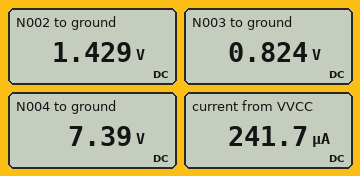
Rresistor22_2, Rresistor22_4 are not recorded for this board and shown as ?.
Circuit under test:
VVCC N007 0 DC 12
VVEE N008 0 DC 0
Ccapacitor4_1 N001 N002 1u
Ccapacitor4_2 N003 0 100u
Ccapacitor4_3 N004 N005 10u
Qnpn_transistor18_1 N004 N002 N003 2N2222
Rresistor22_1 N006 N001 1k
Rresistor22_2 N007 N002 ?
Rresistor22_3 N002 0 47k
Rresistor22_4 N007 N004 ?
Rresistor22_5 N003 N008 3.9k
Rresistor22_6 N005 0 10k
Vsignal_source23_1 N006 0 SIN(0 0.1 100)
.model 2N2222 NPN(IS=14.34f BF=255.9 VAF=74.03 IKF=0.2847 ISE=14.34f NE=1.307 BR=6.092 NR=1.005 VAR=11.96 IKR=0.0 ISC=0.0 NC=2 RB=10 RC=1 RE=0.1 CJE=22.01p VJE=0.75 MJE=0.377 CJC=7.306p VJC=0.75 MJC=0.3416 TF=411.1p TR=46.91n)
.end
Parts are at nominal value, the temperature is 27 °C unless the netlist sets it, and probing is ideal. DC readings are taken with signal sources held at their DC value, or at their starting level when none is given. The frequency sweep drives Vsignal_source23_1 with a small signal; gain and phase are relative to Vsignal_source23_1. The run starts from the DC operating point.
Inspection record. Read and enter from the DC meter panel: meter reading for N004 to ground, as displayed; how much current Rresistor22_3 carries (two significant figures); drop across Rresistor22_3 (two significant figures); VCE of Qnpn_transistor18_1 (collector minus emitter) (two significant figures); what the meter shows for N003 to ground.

7.39 V
30 µA
1.4 V
6.6 V
0.824 V
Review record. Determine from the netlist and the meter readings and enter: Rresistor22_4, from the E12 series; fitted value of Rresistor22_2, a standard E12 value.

22 kΩ
330 kΩ
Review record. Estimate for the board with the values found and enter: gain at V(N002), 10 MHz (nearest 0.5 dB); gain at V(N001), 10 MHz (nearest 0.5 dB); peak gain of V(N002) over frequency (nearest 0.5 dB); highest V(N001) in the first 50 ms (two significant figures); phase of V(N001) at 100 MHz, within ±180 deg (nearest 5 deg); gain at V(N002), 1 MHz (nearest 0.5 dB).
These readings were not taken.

-19.0 dB
-19.0 dB
-0.5 dB
93 mV
-55 deg
-5.5 dB
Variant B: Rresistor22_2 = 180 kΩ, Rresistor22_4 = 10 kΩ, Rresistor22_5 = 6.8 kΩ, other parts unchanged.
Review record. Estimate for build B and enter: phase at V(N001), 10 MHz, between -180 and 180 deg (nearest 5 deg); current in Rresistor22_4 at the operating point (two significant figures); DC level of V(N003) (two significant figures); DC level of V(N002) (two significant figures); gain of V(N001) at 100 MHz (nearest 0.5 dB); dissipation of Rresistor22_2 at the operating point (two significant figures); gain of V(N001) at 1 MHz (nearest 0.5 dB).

-45 deg
260 µA
1.8 V
2.4 V
-28.0 dB
510 µW
-5.0 dB
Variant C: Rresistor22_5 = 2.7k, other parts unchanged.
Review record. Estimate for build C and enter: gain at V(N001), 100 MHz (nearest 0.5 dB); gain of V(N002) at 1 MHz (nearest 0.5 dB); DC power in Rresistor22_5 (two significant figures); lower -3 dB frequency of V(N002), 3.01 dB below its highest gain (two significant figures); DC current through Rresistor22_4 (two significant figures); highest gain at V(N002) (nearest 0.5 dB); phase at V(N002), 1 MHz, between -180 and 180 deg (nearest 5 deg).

-28.0 dB
-8.0 dB
230 µW
15 Hz
290 µA
-1.0 dB
-55 deg
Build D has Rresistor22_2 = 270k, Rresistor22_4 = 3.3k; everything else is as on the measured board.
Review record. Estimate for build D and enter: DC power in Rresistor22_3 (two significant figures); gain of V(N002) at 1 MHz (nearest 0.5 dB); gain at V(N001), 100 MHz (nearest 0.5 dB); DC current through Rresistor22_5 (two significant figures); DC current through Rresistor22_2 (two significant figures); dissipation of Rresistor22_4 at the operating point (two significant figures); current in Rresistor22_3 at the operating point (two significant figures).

61 µW
-2.5 dB
-28.5 dB
280 µA
38 µA
250 µW
36 µA
